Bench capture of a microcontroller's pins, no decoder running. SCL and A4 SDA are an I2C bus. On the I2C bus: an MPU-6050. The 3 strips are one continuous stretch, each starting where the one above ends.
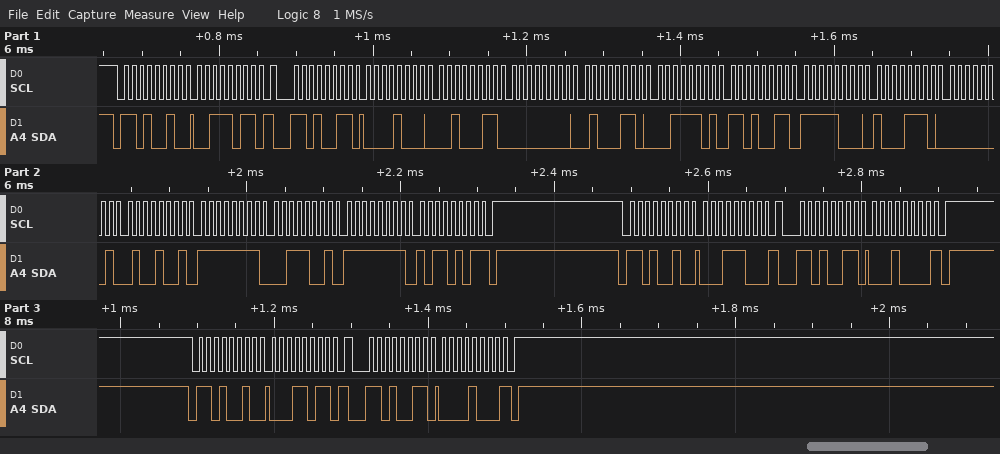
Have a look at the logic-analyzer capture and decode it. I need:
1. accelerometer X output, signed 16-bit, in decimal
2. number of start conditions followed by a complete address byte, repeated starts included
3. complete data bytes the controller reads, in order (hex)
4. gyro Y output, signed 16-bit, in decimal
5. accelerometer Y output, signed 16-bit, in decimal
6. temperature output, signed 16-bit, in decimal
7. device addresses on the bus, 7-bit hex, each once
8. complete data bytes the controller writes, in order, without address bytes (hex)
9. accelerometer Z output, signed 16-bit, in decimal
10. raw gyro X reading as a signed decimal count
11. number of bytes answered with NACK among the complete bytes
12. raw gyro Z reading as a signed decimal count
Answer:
2083
6
08 23 00 46 3D D3 F8 8E 01 49 FF 39 FF B5 10 08
-199
70
-1906
0x69
3B 1C 1B
15827
329
3
-75
